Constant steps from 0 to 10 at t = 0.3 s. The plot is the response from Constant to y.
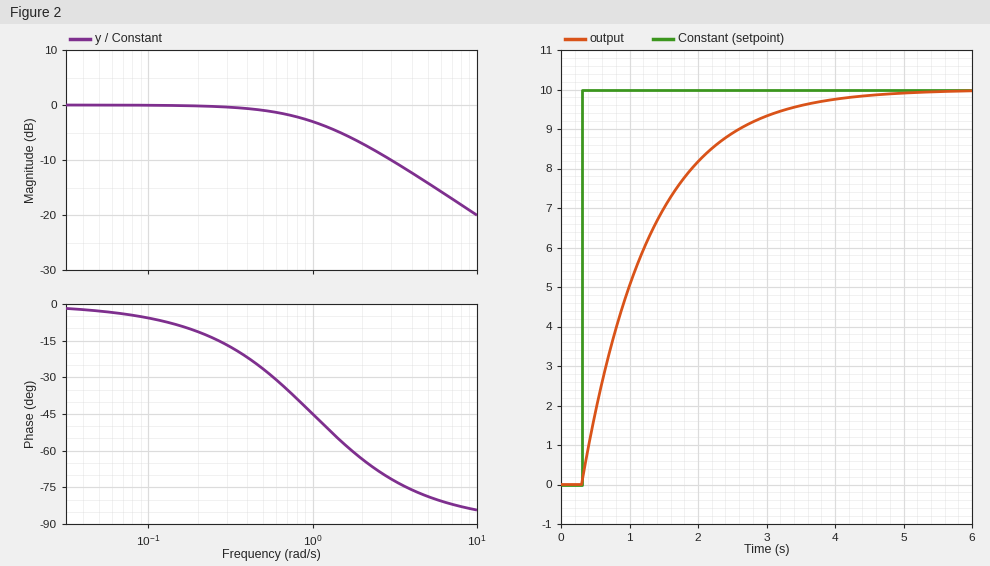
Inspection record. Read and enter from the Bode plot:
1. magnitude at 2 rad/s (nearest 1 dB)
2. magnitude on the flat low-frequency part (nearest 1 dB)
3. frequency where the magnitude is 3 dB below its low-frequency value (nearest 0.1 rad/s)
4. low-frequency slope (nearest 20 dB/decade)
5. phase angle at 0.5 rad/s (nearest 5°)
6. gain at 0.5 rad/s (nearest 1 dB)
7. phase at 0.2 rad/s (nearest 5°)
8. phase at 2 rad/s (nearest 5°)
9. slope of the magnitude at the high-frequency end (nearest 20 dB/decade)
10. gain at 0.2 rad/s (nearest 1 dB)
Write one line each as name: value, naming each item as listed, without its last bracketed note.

magnitude at 2 rad/s: -7 dB
magnitude on the flat low-frequency part: 0 dB
frequency where the magnitude is 3 dB below its low-frequency value: 1.0 rad/s
low-frequency slope: 0 dB/decade
phase angle at 0.5 rad/s: -25°
gain at 0.5 rad/s: -1 dB
phase at 0.2 rad/s: -10°
phase at 2 rad/s: -65°
slope of the magnitude at the high-frequency end: -20 dB/decade
gain at 0.2 rad/s: 0 dB
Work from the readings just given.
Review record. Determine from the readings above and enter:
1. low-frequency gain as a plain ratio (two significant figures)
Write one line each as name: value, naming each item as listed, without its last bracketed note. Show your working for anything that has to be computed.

low-frequency gain as a plain ratio: 10^(0 / 20) = 1.0
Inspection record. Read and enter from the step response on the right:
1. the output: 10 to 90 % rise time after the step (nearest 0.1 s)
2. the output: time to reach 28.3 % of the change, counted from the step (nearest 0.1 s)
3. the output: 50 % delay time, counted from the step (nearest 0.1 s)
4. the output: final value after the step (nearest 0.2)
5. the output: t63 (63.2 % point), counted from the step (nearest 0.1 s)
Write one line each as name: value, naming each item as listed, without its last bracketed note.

the output: 10 to 90 % rise time after the step: 2.2 s
the output: time to reach 28.3 % of the change, counted from the step: 0.3 s
the output: 50 % delay time, counted from the step: 0.7 s
the output: final value after the step: 10.0
the output: t63 (63.2 % point), counted from the step: 1.0 s
